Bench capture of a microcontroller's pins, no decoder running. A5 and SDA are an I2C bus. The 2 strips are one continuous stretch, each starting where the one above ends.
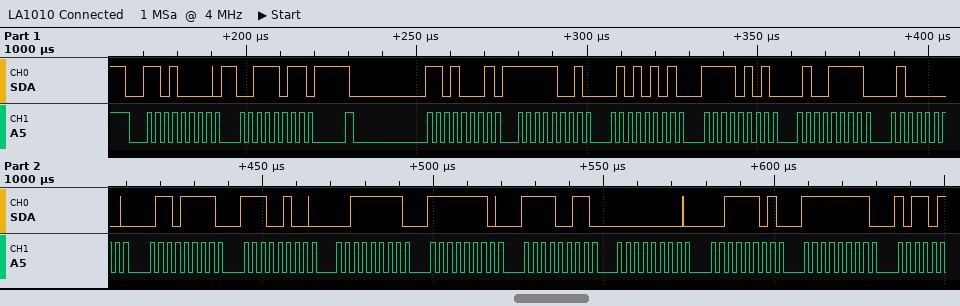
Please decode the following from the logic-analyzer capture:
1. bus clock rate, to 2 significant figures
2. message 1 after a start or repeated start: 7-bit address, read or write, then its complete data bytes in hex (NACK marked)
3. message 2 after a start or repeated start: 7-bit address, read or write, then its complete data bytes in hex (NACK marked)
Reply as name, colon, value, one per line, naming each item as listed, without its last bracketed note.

bus clock rate, to 2 significant figures: 400 kHz
message 1 after a start or repeated start: 7-bit address, read or write, then its complete data bytes in hex: 0x68 write: 3B
message 2 after a start or repeated start: 7-bit address, read or write, then its complete data bytes in hex: 0x68 read: F9 55 F5 4F 40 6F E4 3F FE F3 00 3D FF
